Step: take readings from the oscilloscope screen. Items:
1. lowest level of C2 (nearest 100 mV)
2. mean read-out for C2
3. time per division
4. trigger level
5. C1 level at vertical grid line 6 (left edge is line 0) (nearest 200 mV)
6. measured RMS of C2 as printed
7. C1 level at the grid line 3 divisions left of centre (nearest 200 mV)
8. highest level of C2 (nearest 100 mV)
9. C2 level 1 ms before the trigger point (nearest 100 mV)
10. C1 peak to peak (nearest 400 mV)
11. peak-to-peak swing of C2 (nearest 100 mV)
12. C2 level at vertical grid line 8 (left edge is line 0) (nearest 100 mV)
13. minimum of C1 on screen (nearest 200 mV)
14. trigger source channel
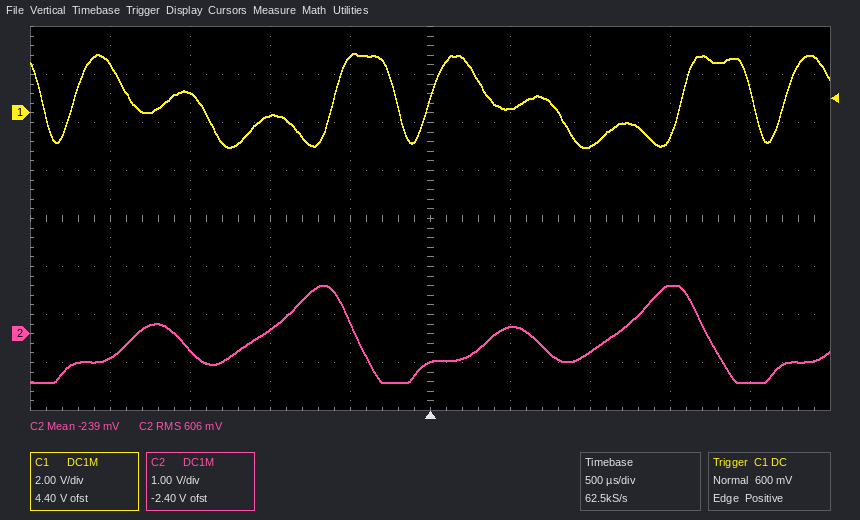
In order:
-1.0 V
-239 mV
500 µs
600 mV
200 mV
606 mV
800 mV
1.0 V
100 mV
4.0 V
2.0 V
1.0 V
-1.4 V
C1
